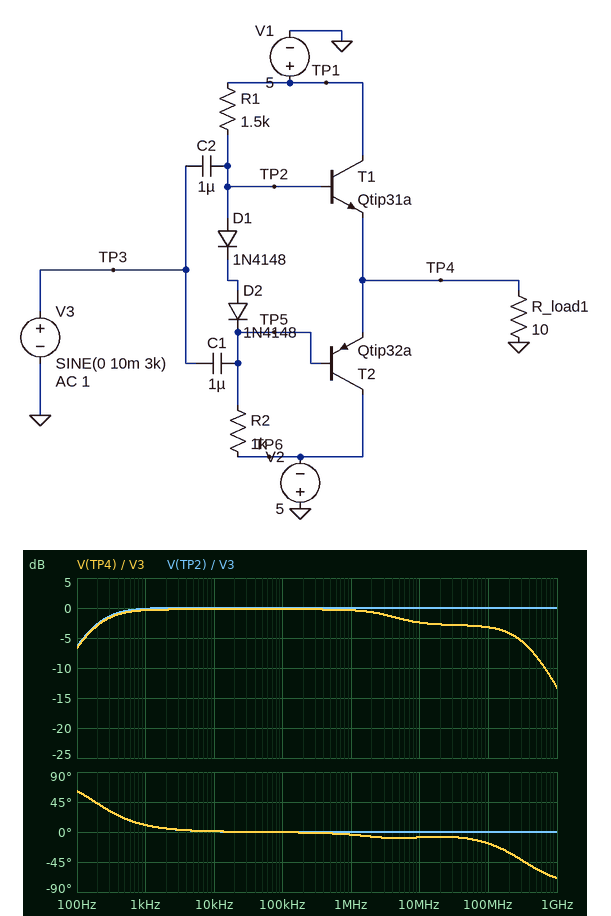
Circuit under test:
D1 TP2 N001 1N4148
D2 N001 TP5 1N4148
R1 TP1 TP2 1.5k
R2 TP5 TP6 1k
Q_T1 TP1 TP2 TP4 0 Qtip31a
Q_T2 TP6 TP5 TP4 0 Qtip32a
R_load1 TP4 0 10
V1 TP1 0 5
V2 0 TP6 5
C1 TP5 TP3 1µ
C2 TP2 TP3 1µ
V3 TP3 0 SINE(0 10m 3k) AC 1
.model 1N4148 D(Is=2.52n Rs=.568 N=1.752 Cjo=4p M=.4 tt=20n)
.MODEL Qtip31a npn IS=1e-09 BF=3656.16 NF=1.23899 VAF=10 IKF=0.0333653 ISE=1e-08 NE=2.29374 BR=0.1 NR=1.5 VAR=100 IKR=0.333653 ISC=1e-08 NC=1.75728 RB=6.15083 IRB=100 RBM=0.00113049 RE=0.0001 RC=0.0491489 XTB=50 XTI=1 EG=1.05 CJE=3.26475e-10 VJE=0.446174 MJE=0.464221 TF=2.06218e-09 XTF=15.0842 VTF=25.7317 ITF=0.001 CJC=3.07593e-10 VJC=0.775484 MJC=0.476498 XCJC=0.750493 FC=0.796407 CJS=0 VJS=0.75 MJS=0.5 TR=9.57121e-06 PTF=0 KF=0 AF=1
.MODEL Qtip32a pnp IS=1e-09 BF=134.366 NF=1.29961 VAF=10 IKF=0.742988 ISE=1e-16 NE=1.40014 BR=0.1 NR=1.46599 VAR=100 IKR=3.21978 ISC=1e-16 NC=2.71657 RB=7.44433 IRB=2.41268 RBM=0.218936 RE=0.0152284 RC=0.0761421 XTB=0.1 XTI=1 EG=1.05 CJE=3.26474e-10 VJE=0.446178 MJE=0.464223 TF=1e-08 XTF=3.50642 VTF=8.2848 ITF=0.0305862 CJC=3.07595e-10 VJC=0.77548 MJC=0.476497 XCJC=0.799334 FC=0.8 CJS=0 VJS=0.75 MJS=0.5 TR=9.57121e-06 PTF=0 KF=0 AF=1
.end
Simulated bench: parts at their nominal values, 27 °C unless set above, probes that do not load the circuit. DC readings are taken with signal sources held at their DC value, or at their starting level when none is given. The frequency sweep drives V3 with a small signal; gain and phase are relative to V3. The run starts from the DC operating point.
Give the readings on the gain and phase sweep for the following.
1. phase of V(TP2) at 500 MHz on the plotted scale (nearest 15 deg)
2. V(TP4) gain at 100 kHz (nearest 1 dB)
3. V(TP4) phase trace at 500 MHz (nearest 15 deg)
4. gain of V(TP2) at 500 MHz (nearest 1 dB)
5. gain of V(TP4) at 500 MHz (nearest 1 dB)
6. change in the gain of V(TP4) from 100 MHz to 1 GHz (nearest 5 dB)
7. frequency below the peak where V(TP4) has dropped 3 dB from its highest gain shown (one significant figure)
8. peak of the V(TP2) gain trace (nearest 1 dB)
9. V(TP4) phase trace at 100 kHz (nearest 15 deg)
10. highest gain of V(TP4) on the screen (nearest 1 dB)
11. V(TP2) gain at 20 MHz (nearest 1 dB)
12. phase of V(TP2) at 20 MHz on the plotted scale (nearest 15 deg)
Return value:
0 deg
0 dB
-60 deg
0 dB
-8 dB
-10 dB
200 Hz
0 dB
0 deg
0 dB
0 dB
0 deg
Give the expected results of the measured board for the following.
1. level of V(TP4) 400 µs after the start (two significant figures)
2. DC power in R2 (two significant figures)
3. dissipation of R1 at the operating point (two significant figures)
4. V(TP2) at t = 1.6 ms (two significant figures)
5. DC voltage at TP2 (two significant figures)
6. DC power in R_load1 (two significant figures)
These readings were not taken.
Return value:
-490 mV
15 mW
16 mW
120 mV
130 mV
25 mW
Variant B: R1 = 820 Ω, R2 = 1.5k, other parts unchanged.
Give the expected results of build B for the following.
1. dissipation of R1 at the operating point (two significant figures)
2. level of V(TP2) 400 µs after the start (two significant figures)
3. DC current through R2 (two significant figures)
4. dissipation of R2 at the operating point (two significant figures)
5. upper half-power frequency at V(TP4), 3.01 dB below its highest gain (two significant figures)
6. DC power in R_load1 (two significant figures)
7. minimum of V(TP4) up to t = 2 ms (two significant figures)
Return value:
13 mW
1.7 V
3.6 mA
20 mW
110 MHz
110 mW
1.0 V
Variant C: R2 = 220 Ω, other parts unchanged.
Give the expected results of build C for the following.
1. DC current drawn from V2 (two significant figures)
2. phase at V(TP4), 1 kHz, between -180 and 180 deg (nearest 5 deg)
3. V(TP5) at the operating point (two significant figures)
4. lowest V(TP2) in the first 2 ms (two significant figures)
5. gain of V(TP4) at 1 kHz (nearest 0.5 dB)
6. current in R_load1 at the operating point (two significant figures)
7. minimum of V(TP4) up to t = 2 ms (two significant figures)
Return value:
370 mA
25 deg
-3.3 V
-2.0 V
-1.0 dB
260 mA
-2.6 V
